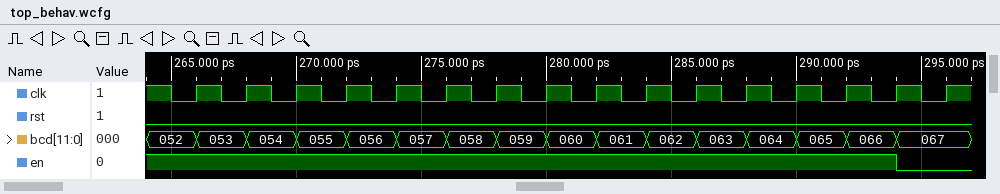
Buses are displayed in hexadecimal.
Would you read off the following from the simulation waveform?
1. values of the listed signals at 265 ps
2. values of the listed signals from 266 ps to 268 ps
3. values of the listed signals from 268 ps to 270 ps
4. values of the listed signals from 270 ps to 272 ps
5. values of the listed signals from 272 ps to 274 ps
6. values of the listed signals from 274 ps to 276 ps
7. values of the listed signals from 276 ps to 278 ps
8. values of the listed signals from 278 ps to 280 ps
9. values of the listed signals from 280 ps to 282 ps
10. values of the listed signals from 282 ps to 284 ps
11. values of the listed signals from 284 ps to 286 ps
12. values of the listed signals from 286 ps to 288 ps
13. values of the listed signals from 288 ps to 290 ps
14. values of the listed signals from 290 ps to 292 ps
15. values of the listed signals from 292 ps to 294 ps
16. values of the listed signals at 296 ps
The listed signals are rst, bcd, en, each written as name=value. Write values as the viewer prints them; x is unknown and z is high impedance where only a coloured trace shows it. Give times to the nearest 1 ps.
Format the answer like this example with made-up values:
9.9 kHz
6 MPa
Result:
rst=0, bcd=052, en=1
rst=0, bcd=053, en=1
rst=0, bcd=054, en=1
rst=0, bcd=055, en=1
rst=0, bcd=056, en=1
rst=0, bcd=057, en=1
rst=0, bcd=058, en=1
rst=0, bcd=059, en=1
rst=0, bcd=060, en=1
rst=0, bcd=061, en=1
rst=0, bcd=062, en=1
rst=0, bcd=063, en=1
rst=0, bcd=064, en=1
rst=0, bcd=065, en=1
rst=0, bcd=066, en=1
rst=0, bcd=067, en=0
